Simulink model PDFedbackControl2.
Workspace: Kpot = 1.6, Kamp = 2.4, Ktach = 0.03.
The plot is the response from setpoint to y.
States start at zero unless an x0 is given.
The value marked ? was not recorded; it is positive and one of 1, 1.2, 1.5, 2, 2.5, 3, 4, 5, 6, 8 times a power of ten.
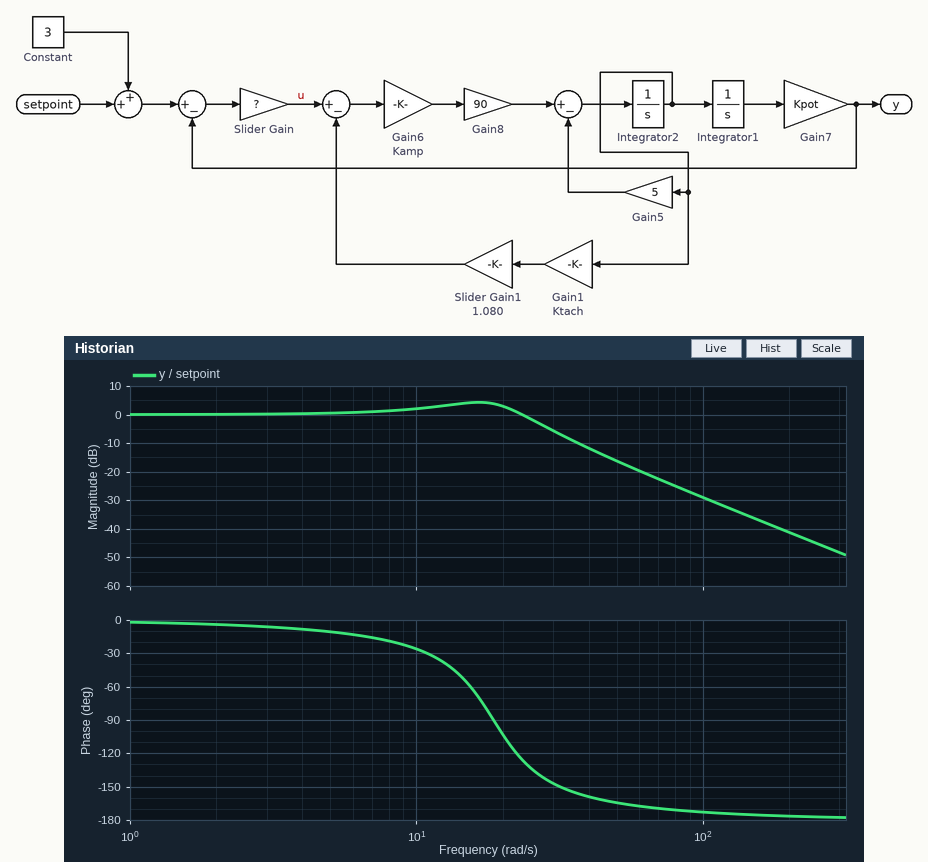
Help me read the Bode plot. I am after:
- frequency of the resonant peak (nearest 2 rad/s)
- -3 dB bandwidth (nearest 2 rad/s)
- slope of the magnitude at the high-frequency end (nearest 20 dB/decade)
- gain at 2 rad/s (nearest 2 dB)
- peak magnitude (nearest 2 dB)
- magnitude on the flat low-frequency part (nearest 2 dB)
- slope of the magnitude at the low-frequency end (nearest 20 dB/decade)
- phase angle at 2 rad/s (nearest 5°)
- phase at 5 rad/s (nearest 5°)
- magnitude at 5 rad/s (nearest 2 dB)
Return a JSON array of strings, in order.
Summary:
["16 rad/s", "26 rad/s", "-40 dB/decade", "0 dB", "4 dB", "0 dB", "0 dB/decade", "-5°", "-10°", "0 dB"]
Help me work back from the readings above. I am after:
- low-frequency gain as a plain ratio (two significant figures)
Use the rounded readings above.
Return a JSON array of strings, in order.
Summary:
["1.0"]
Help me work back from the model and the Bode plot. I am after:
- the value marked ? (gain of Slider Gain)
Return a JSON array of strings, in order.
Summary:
["1"]
